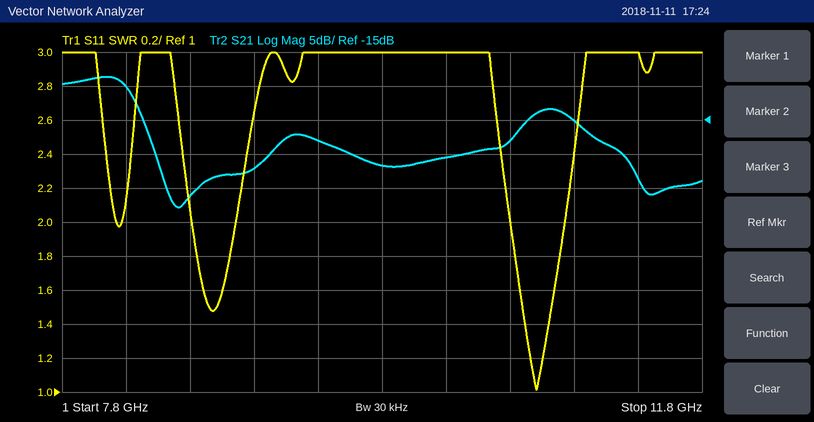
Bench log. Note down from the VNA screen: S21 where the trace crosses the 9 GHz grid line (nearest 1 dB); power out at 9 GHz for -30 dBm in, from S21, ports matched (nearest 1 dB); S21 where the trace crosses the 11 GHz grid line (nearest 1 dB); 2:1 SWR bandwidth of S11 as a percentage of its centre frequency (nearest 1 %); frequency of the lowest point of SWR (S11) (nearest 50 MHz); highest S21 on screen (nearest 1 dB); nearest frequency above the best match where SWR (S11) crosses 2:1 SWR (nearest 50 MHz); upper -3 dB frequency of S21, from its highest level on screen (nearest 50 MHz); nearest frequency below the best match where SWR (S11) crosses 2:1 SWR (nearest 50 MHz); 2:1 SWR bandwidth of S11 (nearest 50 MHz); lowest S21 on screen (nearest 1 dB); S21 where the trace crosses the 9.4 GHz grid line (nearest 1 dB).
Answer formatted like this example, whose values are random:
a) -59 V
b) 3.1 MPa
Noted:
a) -22 dB
b) -52 dBm
c) -15 dB
d) 3 %
e) 10.75 GHz
f) -9 dB
g) 10.95 GHz
h) 8.25 GHz
i) 10.60 GHz
j) 350 MHz
k) -28 dB
l) -18 dB
